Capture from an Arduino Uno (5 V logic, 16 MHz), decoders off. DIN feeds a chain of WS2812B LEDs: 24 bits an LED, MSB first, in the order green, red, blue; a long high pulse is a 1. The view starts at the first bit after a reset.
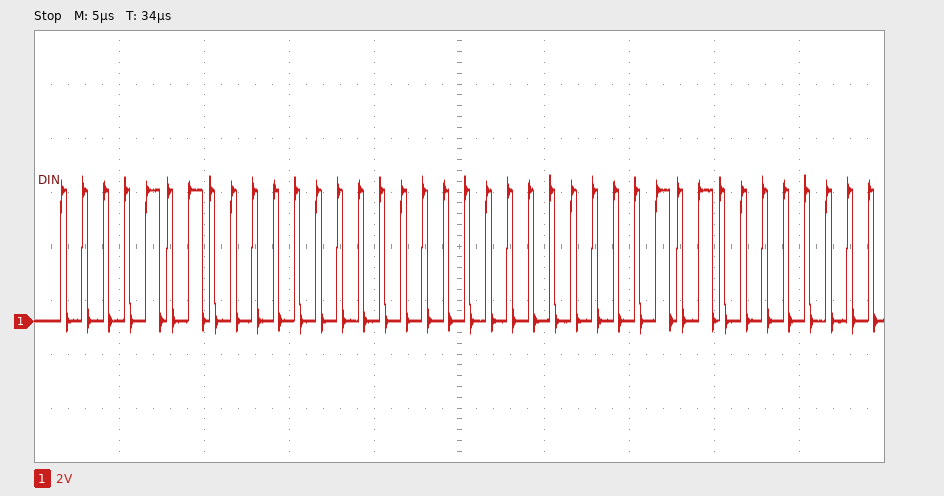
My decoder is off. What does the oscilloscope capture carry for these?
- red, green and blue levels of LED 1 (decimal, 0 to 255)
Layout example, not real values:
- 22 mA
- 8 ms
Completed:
- 0, 10, 0
